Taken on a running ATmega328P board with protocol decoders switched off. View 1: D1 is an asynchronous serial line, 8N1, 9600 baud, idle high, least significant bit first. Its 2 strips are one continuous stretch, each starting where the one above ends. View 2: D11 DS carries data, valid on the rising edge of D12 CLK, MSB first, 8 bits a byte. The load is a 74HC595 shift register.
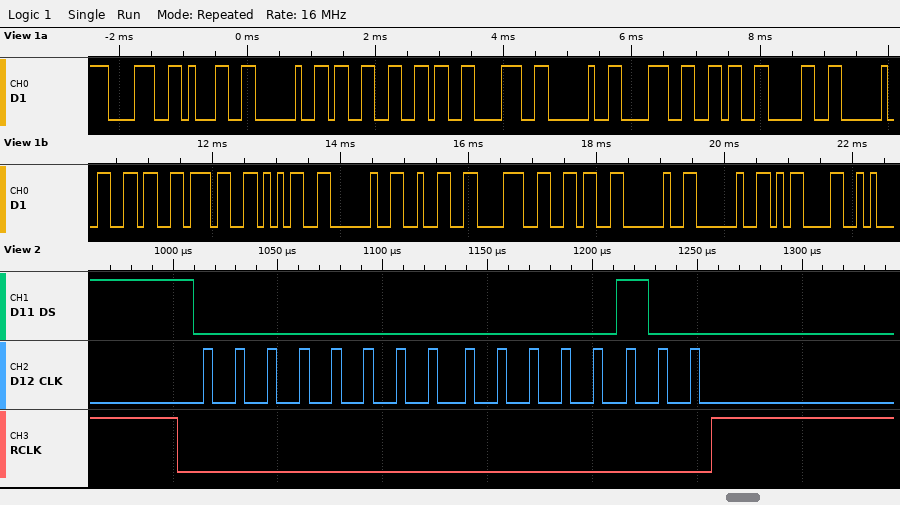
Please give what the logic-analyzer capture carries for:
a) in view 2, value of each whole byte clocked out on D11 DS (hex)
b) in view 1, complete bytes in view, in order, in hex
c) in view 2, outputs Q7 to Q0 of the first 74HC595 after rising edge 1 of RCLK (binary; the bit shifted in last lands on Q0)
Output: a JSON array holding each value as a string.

["00 04", "38 31 20 33 36 38 20 38 36 30 20 36 37 35 20 32 38 36 20 20 0D", "00000100"]
